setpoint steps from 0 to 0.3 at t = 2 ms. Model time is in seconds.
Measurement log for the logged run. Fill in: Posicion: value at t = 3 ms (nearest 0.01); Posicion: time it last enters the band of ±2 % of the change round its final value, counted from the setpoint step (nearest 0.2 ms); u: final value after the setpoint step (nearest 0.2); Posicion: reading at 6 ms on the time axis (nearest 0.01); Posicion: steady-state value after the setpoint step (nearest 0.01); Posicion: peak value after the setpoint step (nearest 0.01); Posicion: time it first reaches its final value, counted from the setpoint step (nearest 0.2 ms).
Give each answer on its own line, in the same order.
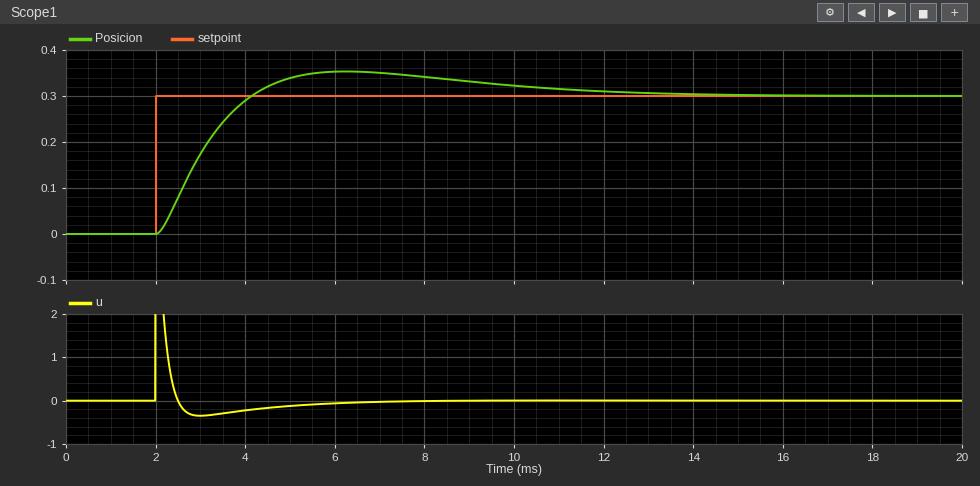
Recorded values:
0.17
11.2 ms
0.0
0.35
0.30
0.35
2.2 ms
